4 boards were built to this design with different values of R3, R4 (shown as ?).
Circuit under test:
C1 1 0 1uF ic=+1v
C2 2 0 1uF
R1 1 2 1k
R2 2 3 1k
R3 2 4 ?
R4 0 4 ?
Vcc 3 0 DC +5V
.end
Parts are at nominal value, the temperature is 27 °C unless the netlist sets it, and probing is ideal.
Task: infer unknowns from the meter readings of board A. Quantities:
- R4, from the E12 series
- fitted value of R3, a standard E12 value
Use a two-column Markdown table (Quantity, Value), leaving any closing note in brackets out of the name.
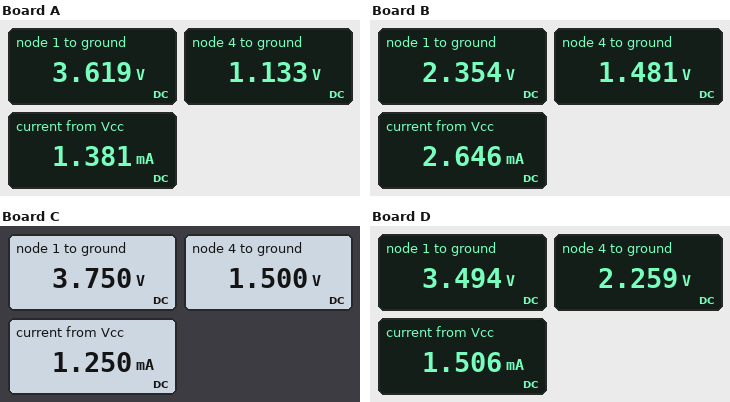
| Quantity | Value |
|---|---|
| R4, from the E12 series | 820 Ω |
| fitted value of R3, a standard E12 value | 1.8 kΩ |
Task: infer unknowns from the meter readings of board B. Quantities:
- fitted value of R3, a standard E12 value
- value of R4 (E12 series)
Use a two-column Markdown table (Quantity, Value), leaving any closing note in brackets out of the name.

| Quantity | Value |
|---|---|
| fitted value of R3, a standard E12 value | 330 Ω |
| value of R4 | 560 Ω |
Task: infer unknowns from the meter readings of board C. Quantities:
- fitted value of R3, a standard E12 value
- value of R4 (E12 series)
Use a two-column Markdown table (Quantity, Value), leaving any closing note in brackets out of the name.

| Quantity | Value |
|---|---|
| fitted value of R3, a standard E12 value | 1.8 kΩ |
| value of R4 | 1.2 kΩ |
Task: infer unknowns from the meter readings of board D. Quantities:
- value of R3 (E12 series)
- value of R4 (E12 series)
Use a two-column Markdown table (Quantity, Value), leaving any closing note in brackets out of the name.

| Quantity | Value |
|---|---|
| value of R3 | 820 Ω |
| value of R4 | 1.5 kΩ |
